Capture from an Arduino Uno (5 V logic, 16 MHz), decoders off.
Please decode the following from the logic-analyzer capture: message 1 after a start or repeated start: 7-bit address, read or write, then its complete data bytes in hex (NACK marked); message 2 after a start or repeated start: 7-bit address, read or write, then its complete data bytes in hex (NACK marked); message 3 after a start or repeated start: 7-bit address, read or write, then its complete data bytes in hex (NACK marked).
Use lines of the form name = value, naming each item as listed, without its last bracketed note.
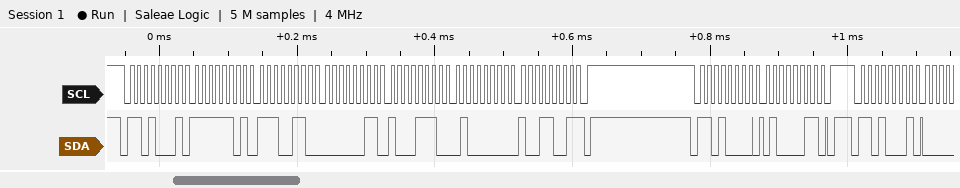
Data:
message 1 after a start or repeated start: 7-bit address, read or write, then its complete data bytes in hex = 0x68 read: FD E6 03 8E 40 99 NACK
message 2 after a start or repeated start: 7-bit address, read or write, then its complete data bytes in hex = 0x68 write: 43
message 3 after a start or repeated start: 7-bit address, read or write, then its complete data bytes in hex = 0x68 read
